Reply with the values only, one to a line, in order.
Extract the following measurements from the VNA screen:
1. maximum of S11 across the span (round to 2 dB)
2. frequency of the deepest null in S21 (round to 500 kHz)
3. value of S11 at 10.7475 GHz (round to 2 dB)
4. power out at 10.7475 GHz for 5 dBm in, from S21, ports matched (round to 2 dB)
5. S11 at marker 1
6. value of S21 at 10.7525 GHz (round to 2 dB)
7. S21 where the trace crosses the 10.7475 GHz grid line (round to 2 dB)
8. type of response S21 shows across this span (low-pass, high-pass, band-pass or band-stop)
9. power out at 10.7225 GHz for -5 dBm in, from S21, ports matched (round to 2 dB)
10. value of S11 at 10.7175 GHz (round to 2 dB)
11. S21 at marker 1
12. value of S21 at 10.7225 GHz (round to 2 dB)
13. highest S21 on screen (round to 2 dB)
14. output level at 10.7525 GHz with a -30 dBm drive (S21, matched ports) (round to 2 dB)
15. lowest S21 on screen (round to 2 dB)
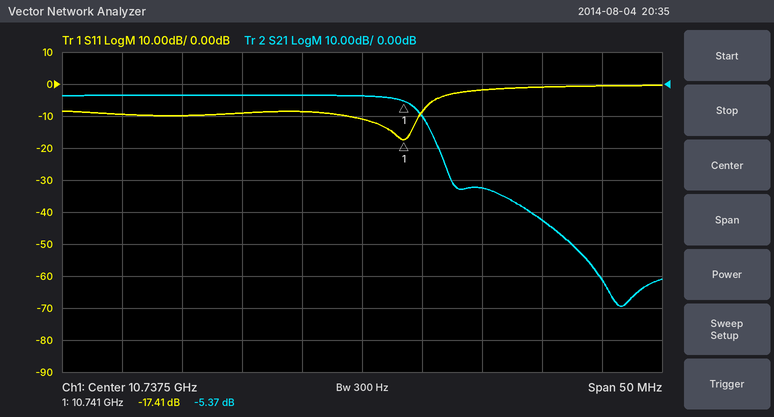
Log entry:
0 dB
10.7590 GHz
-2 dB
-28 dBm
-17.41 dB
-42 dB
-32 dB
low-pass
-8 dBm
-10 dB
-5.37 dB
-4 dB
-4 dB
-72 dBm
-70 dB
